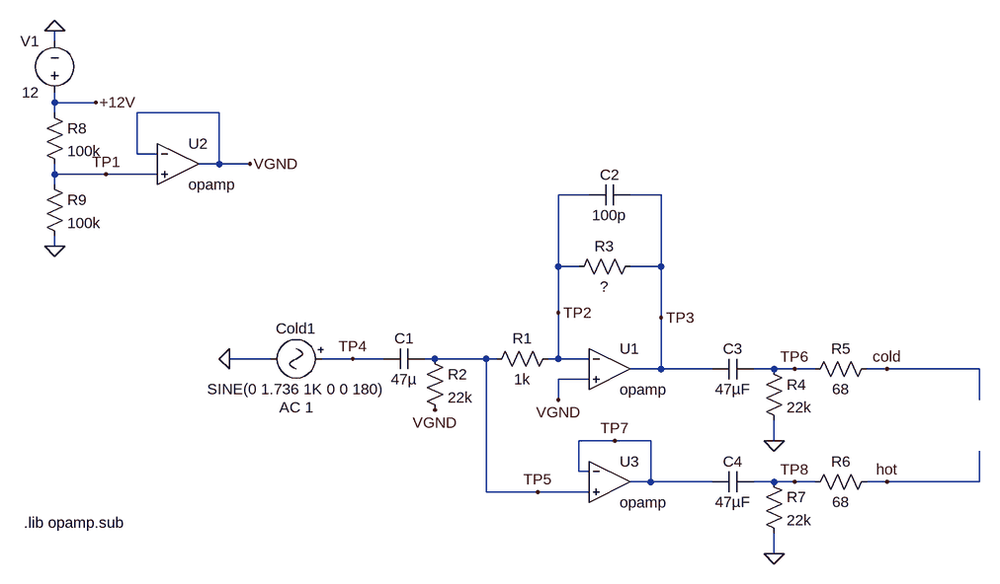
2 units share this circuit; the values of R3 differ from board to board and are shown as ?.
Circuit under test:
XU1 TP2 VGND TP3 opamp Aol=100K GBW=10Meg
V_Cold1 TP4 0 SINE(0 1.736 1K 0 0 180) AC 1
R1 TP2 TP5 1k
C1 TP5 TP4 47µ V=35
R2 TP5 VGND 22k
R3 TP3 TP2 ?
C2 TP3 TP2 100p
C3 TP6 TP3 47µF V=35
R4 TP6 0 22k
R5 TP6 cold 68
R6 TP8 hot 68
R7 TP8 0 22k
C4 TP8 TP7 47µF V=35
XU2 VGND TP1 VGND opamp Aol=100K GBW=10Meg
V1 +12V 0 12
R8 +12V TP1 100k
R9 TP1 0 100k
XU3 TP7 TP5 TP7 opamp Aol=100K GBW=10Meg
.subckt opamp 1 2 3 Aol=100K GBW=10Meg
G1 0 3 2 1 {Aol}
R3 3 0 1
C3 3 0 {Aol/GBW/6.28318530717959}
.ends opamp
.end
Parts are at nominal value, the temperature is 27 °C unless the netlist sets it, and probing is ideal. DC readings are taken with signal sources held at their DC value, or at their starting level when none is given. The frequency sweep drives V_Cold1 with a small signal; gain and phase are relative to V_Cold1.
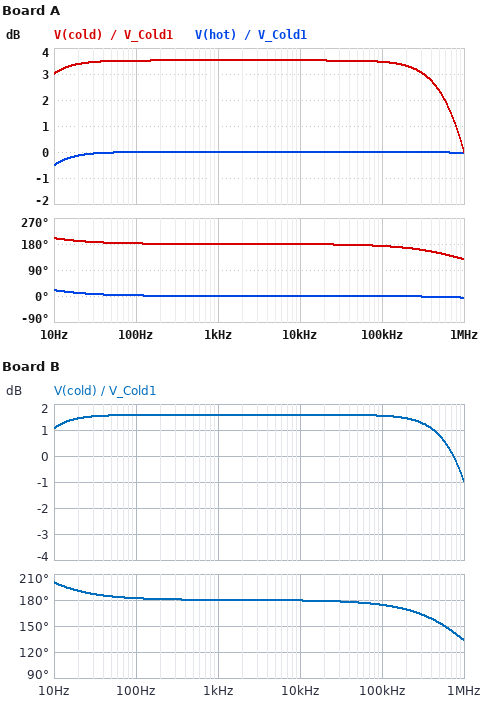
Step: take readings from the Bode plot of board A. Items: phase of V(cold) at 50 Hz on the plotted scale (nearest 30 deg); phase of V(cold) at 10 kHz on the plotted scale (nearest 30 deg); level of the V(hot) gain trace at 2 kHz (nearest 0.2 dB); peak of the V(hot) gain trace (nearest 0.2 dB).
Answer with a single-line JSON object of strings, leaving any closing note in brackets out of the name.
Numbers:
{"phase of V(cold) at 50 Hz on the plotted scale": "180 deg", "phase of V(cold) at 10 kHz on the plotted scale": "180 deg", "level of the V(hot) gain trace at 2 kHz": "0 dB", "peak of the V(hot) gain trace": "0 dB"}
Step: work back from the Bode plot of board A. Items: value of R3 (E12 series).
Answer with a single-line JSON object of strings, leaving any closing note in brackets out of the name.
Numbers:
{"value of R3": "1.5 kΩ"}
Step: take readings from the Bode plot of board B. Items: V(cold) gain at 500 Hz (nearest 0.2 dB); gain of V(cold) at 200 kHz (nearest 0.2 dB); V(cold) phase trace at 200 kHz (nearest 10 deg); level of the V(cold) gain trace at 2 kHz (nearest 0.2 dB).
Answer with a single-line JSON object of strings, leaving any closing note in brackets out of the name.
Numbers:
{"V(cold) gain at 500 Hz": "1.6 dB", "gain of V(cold) at 200 kHz": "1.4 dB", "V(cold) phase trace at 200 kHz": "170 deg", "level of the V(cold) gain trace at 2 kHz": "1.6 dB"}
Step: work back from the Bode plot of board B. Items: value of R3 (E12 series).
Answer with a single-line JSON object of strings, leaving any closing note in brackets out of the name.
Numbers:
{"value of R3": "1.2 kΩ"}
